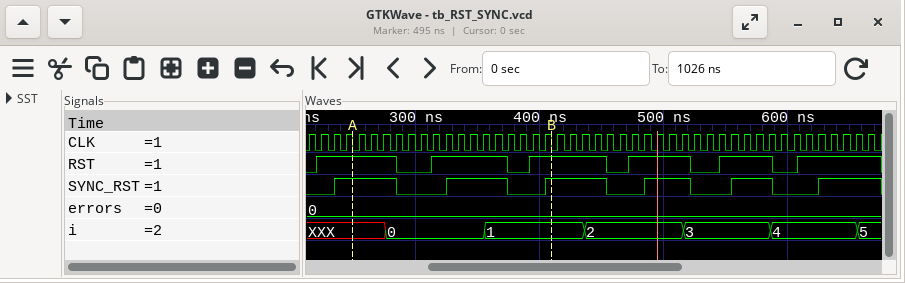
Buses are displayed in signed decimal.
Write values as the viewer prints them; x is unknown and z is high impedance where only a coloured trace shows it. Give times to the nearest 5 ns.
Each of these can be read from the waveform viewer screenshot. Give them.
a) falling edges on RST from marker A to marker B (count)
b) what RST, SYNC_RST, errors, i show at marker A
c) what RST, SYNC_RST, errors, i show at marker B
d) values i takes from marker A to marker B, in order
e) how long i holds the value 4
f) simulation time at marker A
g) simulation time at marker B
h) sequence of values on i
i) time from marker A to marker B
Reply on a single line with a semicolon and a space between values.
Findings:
2; RST=1, SYNC_RST=1, errors=0, i=XXX; RST=1, SYNC_RST=1, errors=0, i=1; XXX, 0, 1; 70 ns; 250 ns; 410 ns; XXX, 0, 1, 2, 3, 4, 5; 160 ns
